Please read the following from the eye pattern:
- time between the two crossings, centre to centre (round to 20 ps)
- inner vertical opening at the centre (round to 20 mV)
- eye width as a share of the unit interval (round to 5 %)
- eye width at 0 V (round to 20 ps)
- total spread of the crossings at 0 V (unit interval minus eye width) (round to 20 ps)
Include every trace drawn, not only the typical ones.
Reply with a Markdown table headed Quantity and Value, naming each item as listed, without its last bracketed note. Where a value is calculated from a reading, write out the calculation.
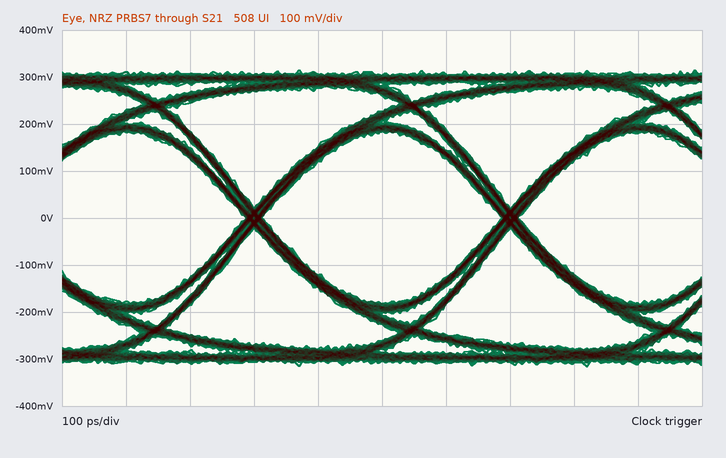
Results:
| Quantity | Value |
|---|---|
| time between the two crossings, centre to centre | 400 ps |
| inner vertical opening at the centre | 360 mV |
| eye width as a share of the unit interval | 380 ps / 400 ps ≈ 95 % |
| eye width at 0 V | 380 ps |
| total spread of the crossings at 0 V (unit interval minus eye width) | 20 ps |
